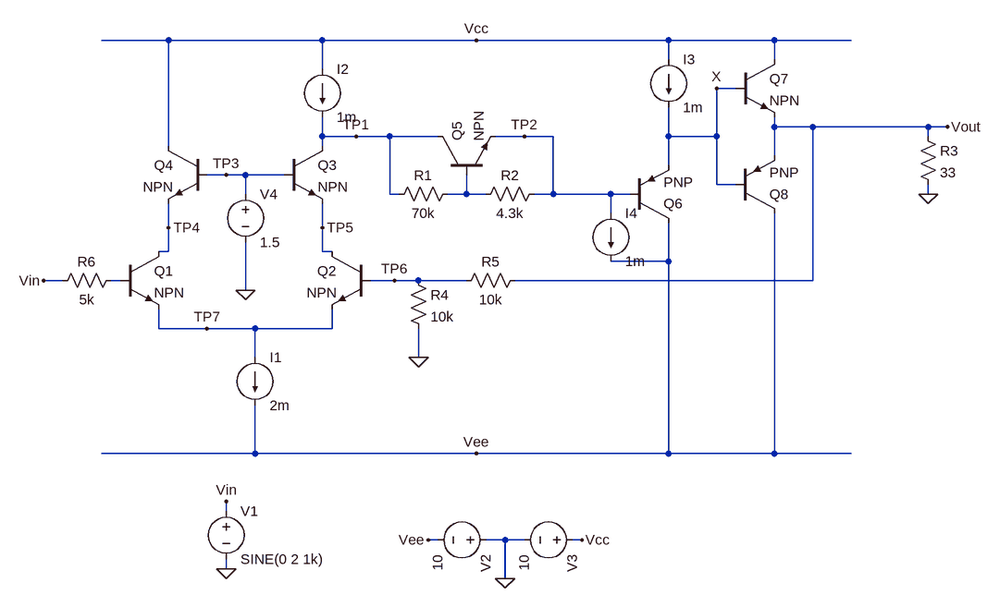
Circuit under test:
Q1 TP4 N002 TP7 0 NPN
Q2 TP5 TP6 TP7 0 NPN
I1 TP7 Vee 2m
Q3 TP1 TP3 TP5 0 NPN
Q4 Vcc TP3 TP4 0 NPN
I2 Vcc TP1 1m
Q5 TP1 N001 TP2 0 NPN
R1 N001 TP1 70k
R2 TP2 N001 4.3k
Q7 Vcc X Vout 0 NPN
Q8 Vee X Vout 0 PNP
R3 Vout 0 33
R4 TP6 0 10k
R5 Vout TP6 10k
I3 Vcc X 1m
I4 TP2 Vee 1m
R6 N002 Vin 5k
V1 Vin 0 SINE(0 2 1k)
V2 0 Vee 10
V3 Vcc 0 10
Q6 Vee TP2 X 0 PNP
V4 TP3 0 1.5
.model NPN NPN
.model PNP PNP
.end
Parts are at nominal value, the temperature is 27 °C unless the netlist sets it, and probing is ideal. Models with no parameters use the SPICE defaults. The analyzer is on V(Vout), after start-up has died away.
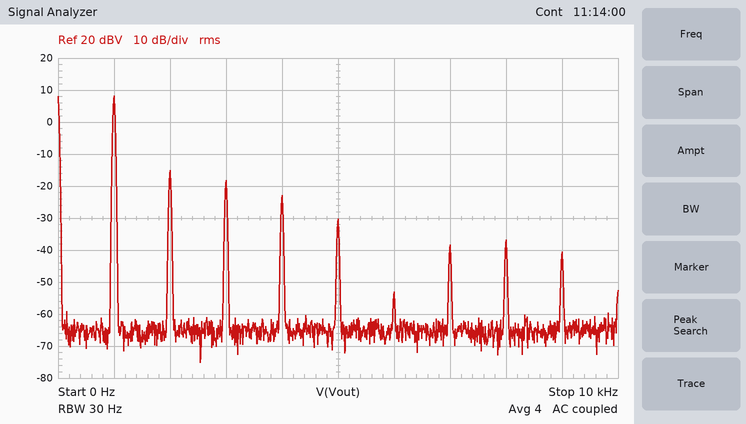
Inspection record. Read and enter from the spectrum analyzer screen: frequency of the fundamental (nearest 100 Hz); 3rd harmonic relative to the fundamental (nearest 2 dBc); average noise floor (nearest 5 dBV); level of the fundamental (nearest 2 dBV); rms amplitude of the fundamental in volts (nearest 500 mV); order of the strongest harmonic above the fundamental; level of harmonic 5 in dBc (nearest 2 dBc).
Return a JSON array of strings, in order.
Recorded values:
["1.0 kHz", "-26 dBc", "-65 dBV", "8 dBV", "2.5 V", "2", "-38 dBc"]
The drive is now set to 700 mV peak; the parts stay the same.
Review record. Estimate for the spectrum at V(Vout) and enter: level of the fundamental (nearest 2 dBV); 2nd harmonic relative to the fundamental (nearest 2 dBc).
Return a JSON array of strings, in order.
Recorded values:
["0 dBV", "-58 dBc"]
